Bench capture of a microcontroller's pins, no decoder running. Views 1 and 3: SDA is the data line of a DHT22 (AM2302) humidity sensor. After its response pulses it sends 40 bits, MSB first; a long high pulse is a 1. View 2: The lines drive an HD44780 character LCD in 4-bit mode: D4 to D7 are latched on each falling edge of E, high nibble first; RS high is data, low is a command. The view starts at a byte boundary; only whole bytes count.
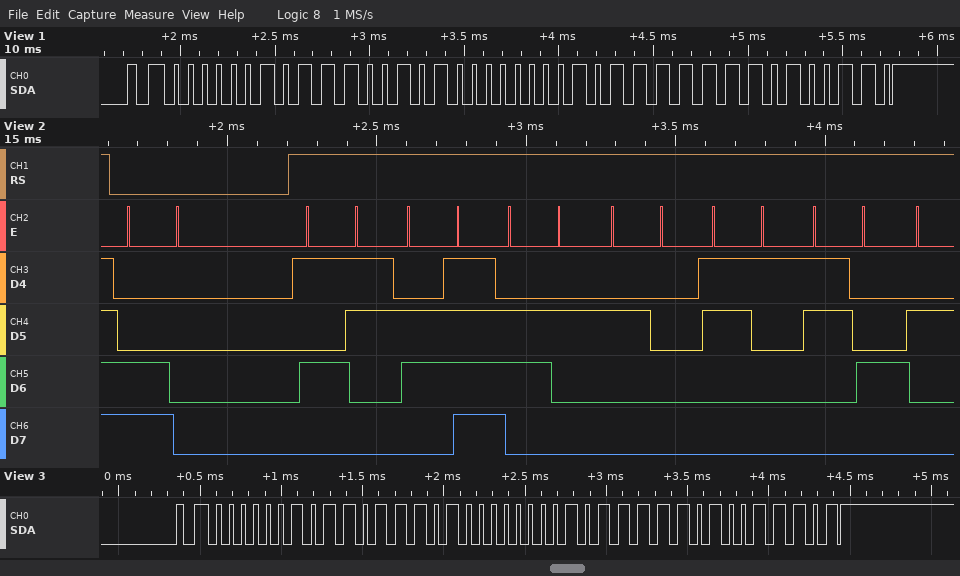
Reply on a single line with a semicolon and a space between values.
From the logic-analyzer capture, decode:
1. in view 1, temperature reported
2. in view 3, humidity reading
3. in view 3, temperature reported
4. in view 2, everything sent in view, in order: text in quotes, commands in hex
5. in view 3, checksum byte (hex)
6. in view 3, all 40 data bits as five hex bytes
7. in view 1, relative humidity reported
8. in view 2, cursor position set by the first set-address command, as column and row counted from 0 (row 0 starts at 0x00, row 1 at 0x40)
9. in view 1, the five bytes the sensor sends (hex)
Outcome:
19.1 °C; 73.3 %; 19.0 °C; 0xC0 "Sob 14"; 0x9D; 02 DD 00 BE 9D; 74.1 %; column 0, row 1; 02 E5 00 BF A6
